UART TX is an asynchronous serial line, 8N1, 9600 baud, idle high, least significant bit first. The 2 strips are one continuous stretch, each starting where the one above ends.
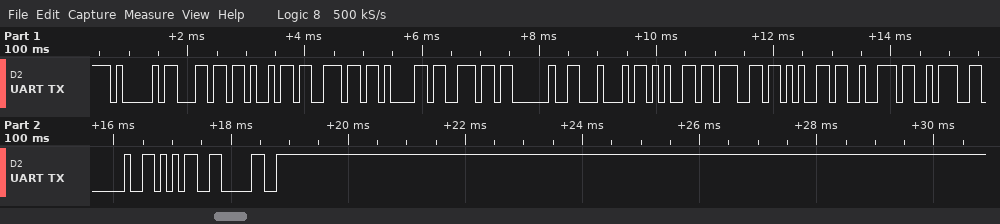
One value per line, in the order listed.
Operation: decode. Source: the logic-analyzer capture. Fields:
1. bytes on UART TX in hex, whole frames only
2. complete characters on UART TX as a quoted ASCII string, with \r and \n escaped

0x41 0x6C 0x69 0x6E 0x61 0x6E 0x20 0x44 0x65 0x67 0x65 0x72 0x3A 0x20 0x35 0x30
"Alinan Deger: 50"
